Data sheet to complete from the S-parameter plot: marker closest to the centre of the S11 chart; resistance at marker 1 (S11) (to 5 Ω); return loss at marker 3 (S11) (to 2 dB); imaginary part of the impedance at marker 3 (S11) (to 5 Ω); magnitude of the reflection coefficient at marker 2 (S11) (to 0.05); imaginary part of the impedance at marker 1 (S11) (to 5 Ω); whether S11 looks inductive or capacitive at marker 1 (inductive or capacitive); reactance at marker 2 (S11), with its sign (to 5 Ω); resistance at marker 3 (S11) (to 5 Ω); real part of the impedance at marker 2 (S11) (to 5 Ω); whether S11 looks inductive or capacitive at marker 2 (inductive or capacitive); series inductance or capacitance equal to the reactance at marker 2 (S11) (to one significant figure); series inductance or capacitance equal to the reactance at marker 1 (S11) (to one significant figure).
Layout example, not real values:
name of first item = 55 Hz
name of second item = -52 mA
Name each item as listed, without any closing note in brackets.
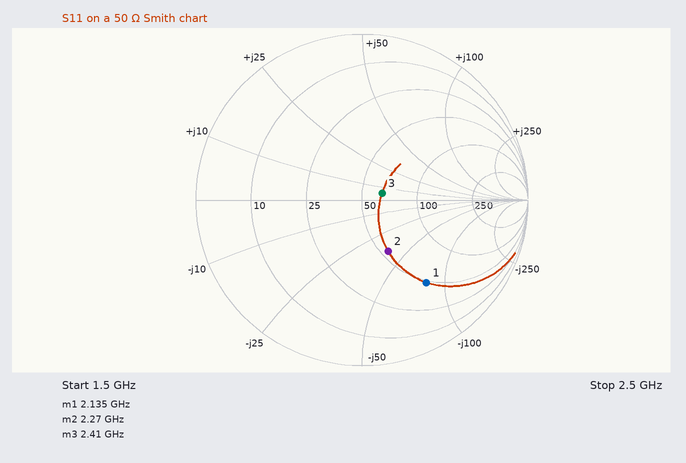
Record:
marker closest to the centre of the S11 chart = marker 3
resistance at marker 1 (S11) = 50 Ω
return loss at marker 3 (S11) = 18 dB
imaginary part of the impedance at marker 3 (S11) = +5 Ω
magnitude of the reflection coefficient at marker 2 (S11) = 0.35
imaginary part of the impedance at marker 1 (S11) = -80 Ω
whether S11 looks inductive or capacitive at marker 1 = capacitive
reactance at marker 2 (S11), with its sign = -40 Ω
resistance at marker 3 (S11) = 65 Ω
real part of the impedance at marker 2 (S11) = 55 Ω
whether S11 looks inductive or capacitive at marker 2 = capacitive
series inductance or capacitance equal to the reactance at marker 2 (S11) = 2 pF
series inductance or capacitance equal to the reactance at marker 1 (S11) = 900 fF
